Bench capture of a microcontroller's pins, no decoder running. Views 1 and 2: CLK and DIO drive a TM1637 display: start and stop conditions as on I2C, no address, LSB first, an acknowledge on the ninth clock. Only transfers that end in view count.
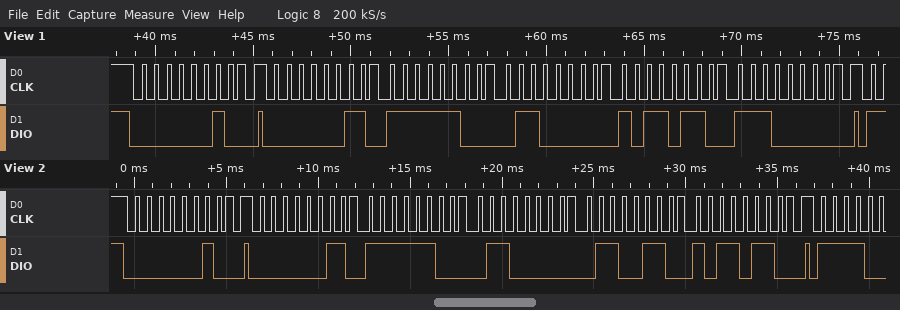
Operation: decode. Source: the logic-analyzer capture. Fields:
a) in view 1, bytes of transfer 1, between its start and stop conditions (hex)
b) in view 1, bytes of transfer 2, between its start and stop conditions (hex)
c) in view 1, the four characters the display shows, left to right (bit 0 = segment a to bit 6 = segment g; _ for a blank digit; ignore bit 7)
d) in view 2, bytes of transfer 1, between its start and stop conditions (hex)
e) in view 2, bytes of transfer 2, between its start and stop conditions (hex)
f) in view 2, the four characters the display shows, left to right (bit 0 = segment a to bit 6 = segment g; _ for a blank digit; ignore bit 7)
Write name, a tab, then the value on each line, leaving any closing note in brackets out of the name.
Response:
in view 1, bytes of transfer 1, between its start and stop conditions	40
in view 1, bytes of transfer 2, between its start and stop conditions	C0 3F 06 6D 07
in view 1, the four characters the display shows, left to right	0157
in view 2, bytes of transfer 1, between its start and stop conditions	40
in view 2, bytes of transfer 2, between its start and stop conditions	C0 3F 06 66 6D
in view 2, the four characters the display shows, left to right	0145
